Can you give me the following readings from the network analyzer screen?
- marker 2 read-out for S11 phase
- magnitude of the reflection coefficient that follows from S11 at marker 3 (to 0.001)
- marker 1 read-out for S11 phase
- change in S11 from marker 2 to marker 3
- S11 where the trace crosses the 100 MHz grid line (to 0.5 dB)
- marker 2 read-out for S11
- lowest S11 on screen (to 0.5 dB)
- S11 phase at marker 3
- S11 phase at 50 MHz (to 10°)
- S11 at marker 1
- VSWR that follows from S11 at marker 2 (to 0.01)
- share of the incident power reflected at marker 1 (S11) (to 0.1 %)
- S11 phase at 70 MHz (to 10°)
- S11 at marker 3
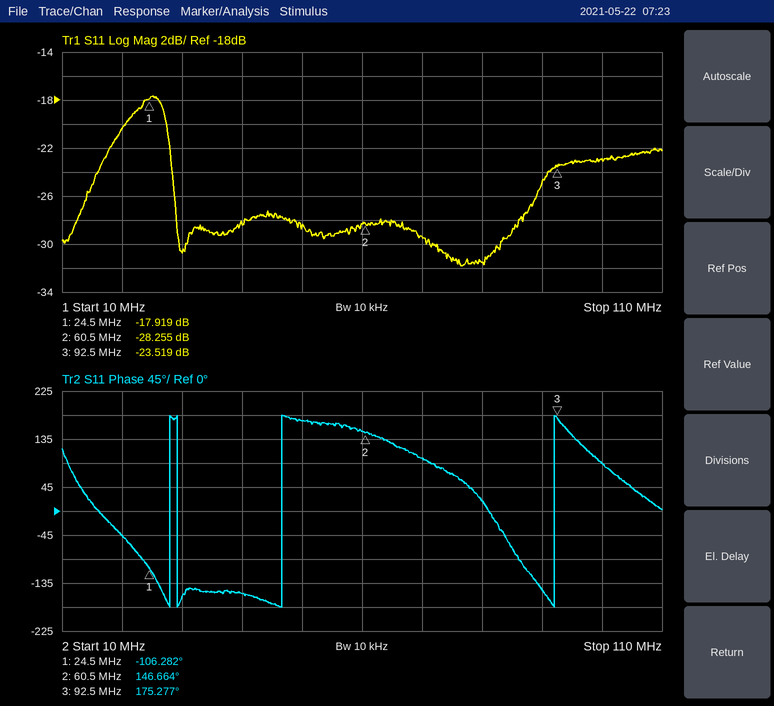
146.664°
0.067
-106.282°
4.736 dB
-23.0 dB
-28.255 dB
-32.0 dB
175.277°
170°
-17.919 dB
1.08
1.6 %
100°
-23.519 dB
